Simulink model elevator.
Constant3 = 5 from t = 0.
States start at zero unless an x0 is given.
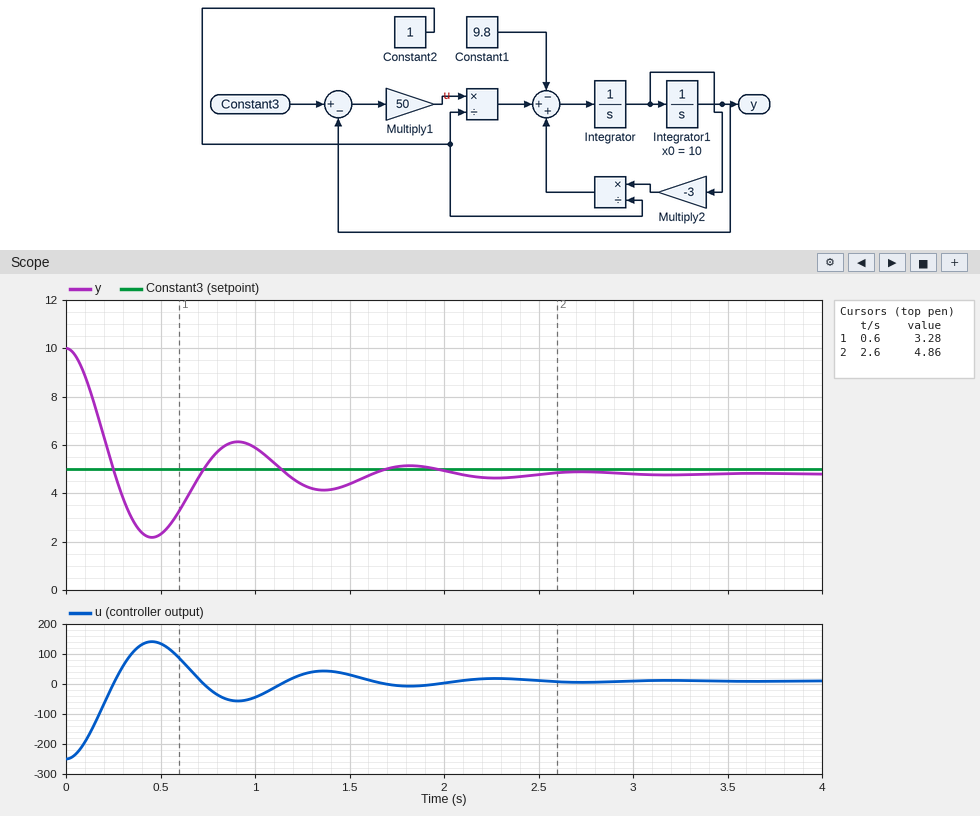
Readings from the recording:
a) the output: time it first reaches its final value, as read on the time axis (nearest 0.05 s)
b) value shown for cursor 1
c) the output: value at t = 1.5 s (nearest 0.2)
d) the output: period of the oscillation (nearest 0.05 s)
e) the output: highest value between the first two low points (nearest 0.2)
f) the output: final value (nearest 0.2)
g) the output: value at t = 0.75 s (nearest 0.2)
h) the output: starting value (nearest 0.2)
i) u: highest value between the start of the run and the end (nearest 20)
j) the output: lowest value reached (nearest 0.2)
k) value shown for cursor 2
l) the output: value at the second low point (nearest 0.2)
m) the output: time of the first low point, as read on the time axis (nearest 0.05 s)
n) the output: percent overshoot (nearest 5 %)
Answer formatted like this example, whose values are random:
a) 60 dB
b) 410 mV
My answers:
a) 0.25 s
b) 3.28
c) 4.4
d) 0.90 s
e) 6.2
f) 4.8
g) 5.2
h) 10.0
i) 140
j) 2.2
k) 4.86
l) 4.2
m) 0.45 s
n) 50 %
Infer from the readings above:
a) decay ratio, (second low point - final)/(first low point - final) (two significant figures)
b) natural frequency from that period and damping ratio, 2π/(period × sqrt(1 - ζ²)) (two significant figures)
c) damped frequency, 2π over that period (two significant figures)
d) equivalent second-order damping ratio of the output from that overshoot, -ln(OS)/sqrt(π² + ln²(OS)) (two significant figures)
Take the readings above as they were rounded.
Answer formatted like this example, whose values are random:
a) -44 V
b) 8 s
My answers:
a) 0.23
b) 7.2 rad/s
c) 7.0 rad/s
d) 0.22
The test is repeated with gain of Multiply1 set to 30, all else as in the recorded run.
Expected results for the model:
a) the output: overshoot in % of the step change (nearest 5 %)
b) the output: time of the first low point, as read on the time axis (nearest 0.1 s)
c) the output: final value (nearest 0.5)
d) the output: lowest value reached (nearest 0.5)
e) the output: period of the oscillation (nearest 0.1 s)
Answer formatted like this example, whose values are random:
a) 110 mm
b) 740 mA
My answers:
a) 40 %
b) 0.6 s
c) 4.5
d) 2.5
e) 1.2 s
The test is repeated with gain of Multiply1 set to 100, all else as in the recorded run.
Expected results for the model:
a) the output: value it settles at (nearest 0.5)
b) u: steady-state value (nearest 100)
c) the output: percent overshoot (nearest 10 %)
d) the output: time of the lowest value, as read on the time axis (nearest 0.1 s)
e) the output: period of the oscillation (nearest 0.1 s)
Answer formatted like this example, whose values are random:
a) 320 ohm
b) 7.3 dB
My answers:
a) 5.0
b) 0
c) 60 %
d) 0.3 s
e) 0.6 s
